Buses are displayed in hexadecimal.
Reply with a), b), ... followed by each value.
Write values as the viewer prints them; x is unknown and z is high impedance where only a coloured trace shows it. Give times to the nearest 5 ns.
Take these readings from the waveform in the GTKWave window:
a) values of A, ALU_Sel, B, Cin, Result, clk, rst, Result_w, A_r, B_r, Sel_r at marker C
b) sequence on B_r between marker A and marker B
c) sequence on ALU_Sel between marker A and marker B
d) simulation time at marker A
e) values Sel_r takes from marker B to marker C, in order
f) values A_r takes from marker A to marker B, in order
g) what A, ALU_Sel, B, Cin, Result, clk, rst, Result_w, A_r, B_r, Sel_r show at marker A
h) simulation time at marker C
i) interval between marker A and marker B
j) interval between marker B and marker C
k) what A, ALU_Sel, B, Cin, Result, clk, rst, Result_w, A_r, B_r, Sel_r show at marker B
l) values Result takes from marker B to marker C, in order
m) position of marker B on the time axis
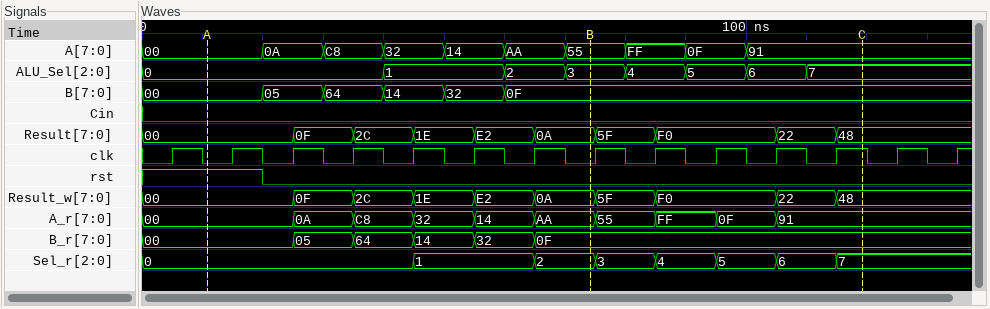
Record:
a) A=91, ALU_Sel=7, B=0F, Cin=0, Result=48, clk=1, rst=0, Result_w=48, A_r=91, B_r=0F, Sel_r=7
b) 00, 05, 64, 14, 32, 0F
c) 0, 1, 2, 3
d) 10 ns
e) 2, 3, 4, 5, 6, 7
f) 00, 0A, C8, 32, 14, AA
g) A=00, ALU_Sel=0, B=00, Cin=0, Result=00, clk=0, rst=1, Result_w=00, A_r=00, B_r=00, Sel_r=0
h) 120 ns
i) 65 ns
j) 45 ns
k) A=55, ALU_Sel=3, B=0F, Cin=0, Result=0A, clk=0, rst=0, Result_w=0A, A_r=AA, B_r=0F, Sel_r=2
l) 0A, 5F, F0, 22, 48
m) 75 ns
